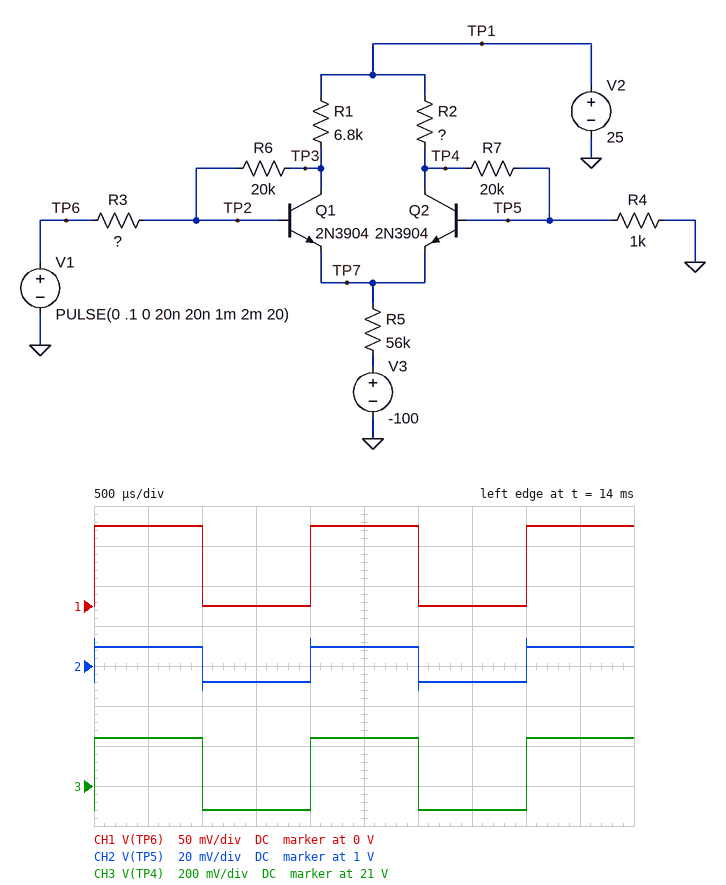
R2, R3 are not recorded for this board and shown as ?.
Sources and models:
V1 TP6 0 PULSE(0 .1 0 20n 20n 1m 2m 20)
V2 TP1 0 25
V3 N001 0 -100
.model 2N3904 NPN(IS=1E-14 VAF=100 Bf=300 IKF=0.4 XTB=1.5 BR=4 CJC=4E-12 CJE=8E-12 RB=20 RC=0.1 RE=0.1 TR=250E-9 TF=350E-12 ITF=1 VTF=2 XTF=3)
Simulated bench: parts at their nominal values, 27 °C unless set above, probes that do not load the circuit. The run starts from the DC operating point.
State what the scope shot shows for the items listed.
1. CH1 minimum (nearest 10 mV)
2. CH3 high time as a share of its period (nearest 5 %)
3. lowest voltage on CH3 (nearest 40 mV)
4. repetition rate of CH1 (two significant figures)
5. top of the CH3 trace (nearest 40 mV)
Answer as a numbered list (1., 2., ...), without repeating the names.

1. 0 V
2. 50 %
3. 20.88 V
4. 500 Hz
5. 21.24 V
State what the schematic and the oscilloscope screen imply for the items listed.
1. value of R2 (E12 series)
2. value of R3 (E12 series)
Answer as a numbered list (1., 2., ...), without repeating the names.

1. 2.2 kΩ
2. 1.5 kΩ
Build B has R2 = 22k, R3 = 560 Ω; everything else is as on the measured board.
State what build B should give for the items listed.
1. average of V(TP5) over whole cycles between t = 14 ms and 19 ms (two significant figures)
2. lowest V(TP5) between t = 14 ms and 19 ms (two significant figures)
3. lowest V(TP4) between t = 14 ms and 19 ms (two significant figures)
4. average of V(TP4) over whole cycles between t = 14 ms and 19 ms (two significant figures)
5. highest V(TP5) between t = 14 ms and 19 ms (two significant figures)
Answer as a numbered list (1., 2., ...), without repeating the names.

1. 350 mV
2. 310 mV
3. 6.6 V
4. 7.3 V
5. 380 mV
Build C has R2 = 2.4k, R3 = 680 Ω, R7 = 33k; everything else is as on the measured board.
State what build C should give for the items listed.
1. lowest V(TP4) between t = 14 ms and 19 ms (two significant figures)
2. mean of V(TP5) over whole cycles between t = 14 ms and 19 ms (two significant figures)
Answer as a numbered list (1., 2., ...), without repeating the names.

1. 20 V
2. 600 mV
